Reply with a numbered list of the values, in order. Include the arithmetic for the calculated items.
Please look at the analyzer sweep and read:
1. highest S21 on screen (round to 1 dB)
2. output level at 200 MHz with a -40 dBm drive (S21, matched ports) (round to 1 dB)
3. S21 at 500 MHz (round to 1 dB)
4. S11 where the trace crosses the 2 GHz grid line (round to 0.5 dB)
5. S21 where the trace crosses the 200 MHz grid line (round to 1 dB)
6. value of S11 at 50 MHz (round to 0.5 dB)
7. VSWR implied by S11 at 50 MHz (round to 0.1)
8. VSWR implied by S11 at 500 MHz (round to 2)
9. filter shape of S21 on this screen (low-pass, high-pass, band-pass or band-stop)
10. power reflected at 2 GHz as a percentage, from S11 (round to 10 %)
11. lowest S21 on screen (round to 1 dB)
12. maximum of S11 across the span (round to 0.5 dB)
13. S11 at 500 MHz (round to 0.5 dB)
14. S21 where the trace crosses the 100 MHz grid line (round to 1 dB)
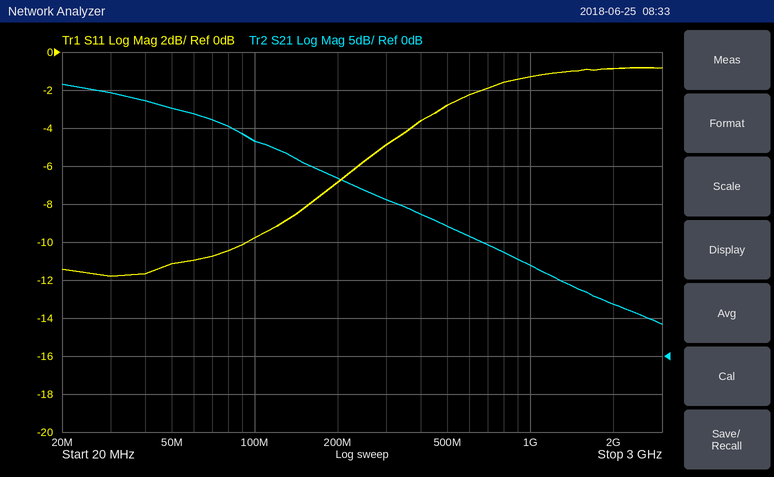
1. 36 dB
2. -40 dBm + (23 dB) = -17 dBm
3. 17 dB
4. -1.0 dB
5. 23 dB
6. -11.0 dB
7. |Γ| = 10^(-11/20) = 0.2818; VSWR = (1 + 0.2818)/(1 − 0.2818) ≈ 1.8
8. |Γ| = 10^(-3/20) = 0.7079; VSWR = (1 + 0.7079)/(1 − 0.7079) ≈ 6
9. low-pass
10. 10^(-1/10) ≈ 79.4 %, so 80 % to the nearest 10 %
11. 4 dB
12. -1.0 dB
13. -3.0 dB
14. 28 dB
